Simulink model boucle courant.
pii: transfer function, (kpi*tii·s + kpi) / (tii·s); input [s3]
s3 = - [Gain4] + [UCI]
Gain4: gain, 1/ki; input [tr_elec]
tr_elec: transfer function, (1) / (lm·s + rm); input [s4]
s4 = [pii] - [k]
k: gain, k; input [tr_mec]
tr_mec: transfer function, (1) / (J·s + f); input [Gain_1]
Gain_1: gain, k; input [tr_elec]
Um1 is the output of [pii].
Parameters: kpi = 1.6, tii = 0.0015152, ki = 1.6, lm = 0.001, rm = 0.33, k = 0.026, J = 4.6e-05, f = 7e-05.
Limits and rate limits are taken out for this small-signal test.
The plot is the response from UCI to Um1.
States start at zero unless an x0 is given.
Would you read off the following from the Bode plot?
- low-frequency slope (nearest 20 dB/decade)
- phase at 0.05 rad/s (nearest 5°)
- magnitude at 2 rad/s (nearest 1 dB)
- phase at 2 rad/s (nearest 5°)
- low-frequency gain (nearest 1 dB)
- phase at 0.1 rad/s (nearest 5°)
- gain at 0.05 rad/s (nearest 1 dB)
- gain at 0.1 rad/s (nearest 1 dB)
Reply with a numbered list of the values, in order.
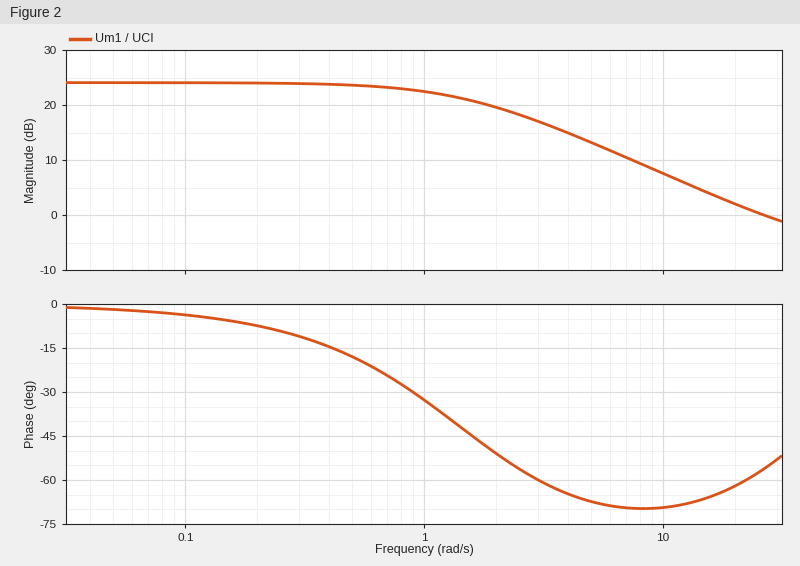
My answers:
1. 0 dB/decade
2. 0°
3. 20 dB
4. -50°
5. 24 dB
6. -5°
7. 24 dB
8. 24 dB
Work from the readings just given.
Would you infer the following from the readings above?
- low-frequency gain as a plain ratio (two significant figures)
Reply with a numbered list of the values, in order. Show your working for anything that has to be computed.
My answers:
1. 10^(24 / 20) = 16
